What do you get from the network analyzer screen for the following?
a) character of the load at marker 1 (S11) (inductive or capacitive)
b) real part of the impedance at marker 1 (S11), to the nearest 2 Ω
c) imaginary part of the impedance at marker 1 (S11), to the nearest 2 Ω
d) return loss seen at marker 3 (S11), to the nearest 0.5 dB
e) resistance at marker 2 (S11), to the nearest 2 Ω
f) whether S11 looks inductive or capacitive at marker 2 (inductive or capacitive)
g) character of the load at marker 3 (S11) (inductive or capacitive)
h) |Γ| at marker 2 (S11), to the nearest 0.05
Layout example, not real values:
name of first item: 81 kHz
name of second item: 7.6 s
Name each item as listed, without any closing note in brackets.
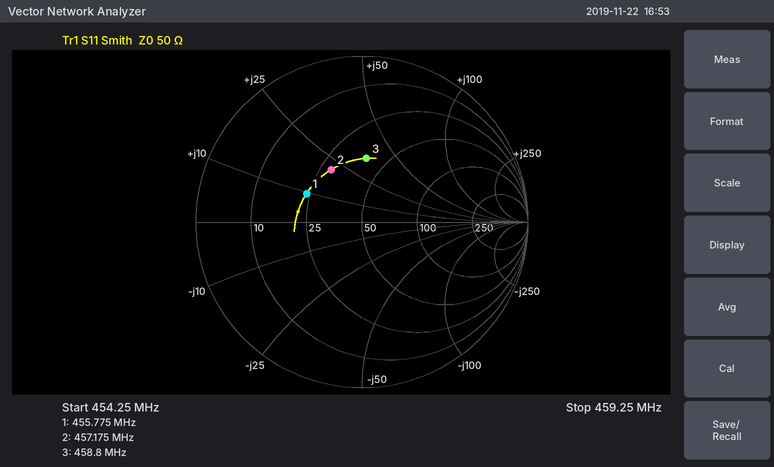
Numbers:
character of the load at marker 1 (S11): inductive
real part of the impedance at marker 1 (S11), to the nearest 2 Ω: 24 Ω
imaginary part of the impedance at marker 1 (S11), to the nearest 2 Ω: +10 Ω
return loss seen at marker 3 (S11), to the nearest 0.5 dB: 8.5 dB
resistance at marker 2 (S11), to the nearest 2 Ω: 28 Ω
whether S11 looks inductive or capacitive at marker 2: inductive
character of the load at marker 3 (S11): inductive
|Γ| at marker 2 (S11), to the nearest 0.05: 0.35
